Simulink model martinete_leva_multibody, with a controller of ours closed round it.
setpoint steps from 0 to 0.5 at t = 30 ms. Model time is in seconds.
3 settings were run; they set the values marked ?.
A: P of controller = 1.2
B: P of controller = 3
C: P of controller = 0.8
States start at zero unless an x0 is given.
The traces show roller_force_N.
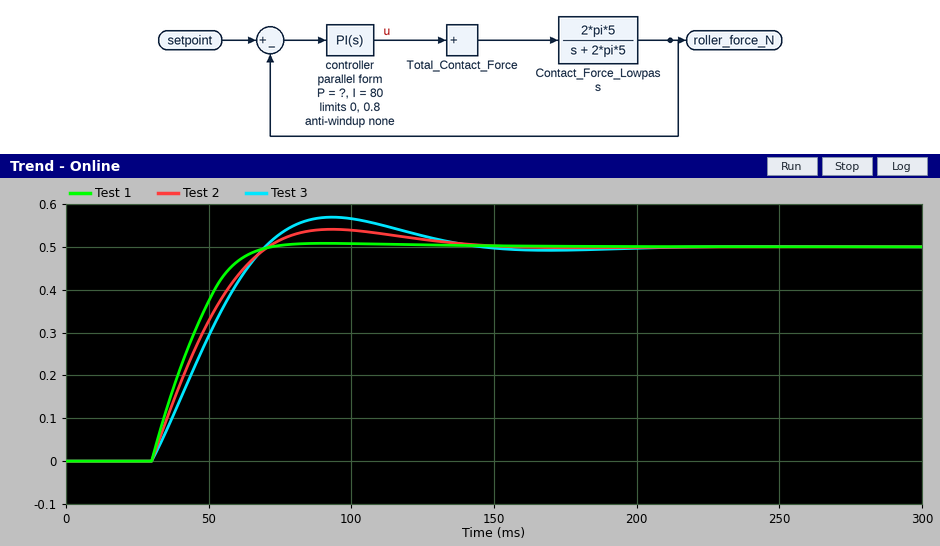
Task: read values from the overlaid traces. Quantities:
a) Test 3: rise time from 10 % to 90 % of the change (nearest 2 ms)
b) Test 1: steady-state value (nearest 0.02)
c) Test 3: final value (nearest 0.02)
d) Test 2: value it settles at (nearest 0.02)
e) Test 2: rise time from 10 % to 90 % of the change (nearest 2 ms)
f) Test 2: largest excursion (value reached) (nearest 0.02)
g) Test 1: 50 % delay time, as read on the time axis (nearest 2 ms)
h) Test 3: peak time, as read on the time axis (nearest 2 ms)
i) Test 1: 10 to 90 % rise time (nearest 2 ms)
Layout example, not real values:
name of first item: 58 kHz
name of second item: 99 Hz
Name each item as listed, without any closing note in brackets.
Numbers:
Test 3: rise time from 10 % to 90 % of the change: 30 ms
Test 1: steady-state value: 0.50
Test 3: final value: 0.50
Test 2: value it settles at: 0.50
Test 2: rise time from 10 % to 90 % of the change: 30 ms
Test 2: largest excursion (value reached): 0.54
Test 1: 50 % delay time, as read on the time axis: 42 ms
Test 3: peak time, as read on the time axis: 94 ms
Test 1: 10 to 90 % rise time: 26 ms
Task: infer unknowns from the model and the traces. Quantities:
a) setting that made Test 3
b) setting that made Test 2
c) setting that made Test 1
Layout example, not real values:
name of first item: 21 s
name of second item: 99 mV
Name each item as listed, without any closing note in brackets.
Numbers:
setting that made Test 3: C
setting that made Test 2: A
setting that made Test 1: B
